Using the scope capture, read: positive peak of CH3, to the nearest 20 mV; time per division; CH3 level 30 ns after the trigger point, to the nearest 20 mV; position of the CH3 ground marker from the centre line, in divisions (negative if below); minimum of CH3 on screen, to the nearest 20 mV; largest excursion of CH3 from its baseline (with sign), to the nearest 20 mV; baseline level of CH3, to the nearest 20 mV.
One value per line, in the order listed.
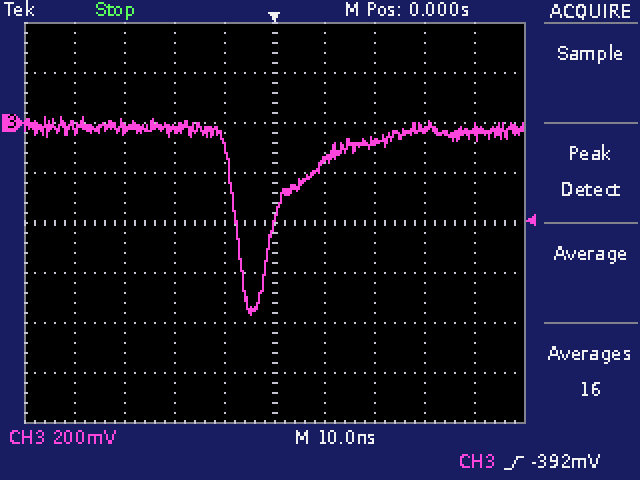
20 mV
10 ns
-20 mV
+2.0 div
-760 mV
-740 mV
-20 mV
